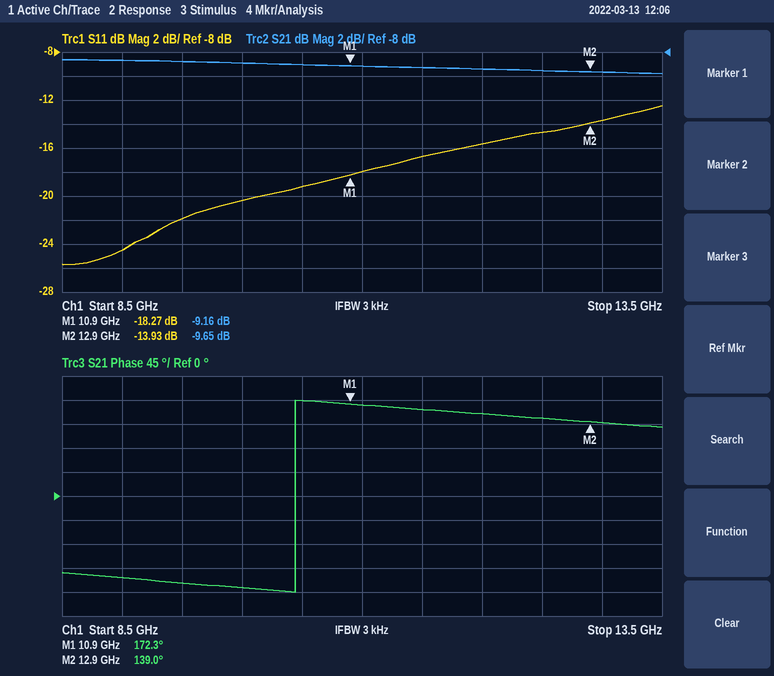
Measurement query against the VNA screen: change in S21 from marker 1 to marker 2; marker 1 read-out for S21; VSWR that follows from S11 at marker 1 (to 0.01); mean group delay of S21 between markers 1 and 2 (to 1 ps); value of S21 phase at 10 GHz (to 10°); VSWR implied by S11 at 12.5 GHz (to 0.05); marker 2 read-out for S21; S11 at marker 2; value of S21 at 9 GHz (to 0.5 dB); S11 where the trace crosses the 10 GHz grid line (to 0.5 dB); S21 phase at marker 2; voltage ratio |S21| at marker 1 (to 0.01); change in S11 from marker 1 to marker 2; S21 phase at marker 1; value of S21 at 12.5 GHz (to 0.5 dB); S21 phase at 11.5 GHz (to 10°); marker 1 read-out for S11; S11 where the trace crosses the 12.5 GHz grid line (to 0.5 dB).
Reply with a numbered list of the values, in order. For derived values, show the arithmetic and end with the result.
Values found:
1. -9.65 − (-9.16) = -0.49 dB
2. -9.16 dB
3. (1 + 0.1220)/(1 − 0.1220) ≈ 1.28
4. −(139° − (172.3°))/(360° × 2 GHz) ≈ 46 ps
5. -170°
6. |Γ| = 10^(-14.5/20) = 0.1884; VSWR = (1 + 0.1884)/(1 − 0.1884) ≈ 1.46, so 1.45 to the nearest 0.05
7. -9.65 dB
8. -13.93 dB
9. -8.5 dB
10. -20.5 dB
11. 139.0°
12. 10^(-9.16/20) ≈ 0.35
13. -13.93 − (-18.27) = 4.34 dB
14. 172.3°
15. -9.5 dB
16. 160°
17. -18.27 dB
18. -14.5 dB
